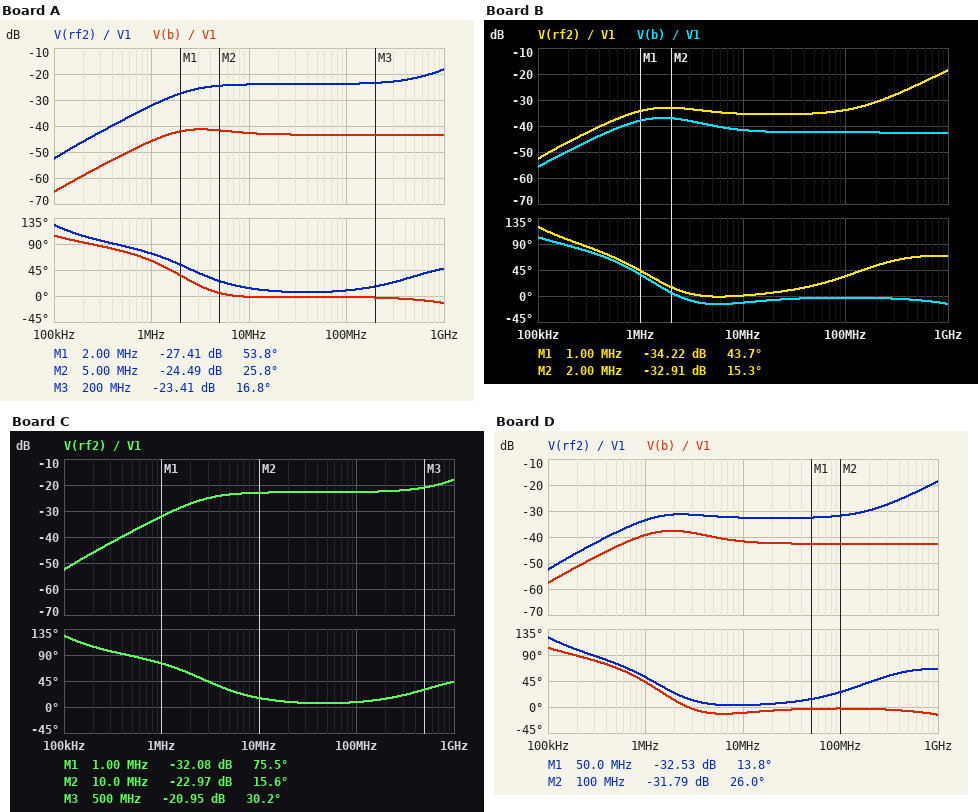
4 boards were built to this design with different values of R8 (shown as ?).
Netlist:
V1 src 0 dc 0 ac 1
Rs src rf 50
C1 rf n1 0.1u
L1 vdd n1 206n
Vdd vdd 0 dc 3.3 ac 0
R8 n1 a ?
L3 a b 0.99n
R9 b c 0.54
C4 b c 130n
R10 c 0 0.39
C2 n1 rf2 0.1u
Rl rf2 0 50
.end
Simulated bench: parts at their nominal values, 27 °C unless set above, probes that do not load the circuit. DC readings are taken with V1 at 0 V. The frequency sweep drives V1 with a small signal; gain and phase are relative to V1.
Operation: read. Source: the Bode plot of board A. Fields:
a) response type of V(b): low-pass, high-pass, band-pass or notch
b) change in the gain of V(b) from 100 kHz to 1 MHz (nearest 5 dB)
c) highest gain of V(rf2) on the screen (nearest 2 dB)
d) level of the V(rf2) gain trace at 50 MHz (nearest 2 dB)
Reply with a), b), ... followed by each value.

a) high-pass
b) 20 dB
c) -18 dB
d) -24 dB
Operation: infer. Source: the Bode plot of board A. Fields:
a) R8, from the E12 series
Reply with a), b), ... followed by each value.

a) 3.3 Ω
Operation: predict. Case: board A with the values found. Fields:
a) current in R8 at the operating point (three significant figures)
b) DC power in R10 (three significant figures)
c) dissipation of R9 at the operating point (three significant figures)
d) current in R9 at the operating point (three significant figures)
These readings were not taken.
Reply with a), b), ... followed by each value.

a) 780 mA
b) 237 mW
c) 329 mW
d) 780 mA
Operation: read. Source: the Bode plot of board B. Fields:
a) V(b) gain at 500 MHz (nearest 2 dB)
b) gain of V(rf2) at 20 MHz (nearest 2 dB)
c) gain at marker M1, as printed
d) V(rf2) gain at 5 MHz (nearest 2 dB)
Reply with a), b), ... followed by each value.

a) -42 dB
b) -36 dB
c) -34.22 dB
d) -34 dB
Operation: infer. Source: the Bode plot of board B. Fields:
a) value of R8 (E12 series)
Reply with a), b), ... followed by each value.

a) 0.47 Ω
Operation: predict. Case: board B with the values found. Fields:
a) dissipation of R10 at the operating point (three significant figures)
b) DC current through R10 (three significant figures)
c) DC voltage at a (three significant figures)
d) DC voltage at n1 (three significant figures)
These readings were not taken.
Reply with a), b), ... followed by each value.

a) 2.17 W
b) 2.36 A
c) 2.19 V
d) 3.30 V
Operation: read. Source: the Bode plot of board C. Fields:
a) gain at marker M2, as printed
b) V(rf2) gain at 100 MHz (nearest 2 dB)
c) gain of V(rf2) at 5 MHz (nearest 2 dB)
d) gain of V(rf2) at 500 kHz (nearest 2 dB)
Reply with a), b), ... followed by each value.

a) -22.97 dB
b) -22 dB
c) -24 dB
d) -38 dB
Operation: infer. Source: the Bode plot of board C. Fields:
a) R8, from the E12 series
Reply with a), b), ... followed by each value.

a) 3.9 Ω
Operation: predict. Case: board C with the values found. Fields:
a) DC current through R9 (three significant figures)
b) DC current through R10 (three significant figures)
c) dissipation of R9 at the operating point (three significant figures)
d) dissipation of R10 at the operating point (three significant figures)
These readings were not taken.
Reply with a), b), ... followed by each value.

a) 683 mA
b) 683 mA
c) 252 mW
d) 182 mW
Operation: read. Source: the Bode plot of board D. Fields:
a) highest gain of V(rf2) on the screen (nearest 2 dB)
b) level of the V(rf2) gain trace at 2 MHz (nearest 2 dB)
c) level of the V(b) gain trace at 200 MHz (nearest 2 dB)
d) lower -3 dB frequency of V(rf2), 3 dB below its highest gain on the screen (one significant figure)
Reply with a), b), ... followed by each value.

a) -18 dB
b) -32 dB
c) -42 dB
d) 700 MHz
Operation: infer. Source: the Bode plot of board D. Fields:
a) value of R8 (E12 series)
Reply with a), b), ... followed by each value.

a) 0.82 Ω
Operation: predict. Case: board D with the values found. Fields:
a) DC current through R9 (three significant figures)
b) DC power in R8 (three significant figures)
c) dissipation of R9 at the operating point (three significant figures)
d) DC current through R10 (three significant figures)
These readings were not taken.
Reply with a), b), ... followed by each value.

a) 1.89 A
b) 2.92 W
c) 1.92 W
d) 1.89 A
